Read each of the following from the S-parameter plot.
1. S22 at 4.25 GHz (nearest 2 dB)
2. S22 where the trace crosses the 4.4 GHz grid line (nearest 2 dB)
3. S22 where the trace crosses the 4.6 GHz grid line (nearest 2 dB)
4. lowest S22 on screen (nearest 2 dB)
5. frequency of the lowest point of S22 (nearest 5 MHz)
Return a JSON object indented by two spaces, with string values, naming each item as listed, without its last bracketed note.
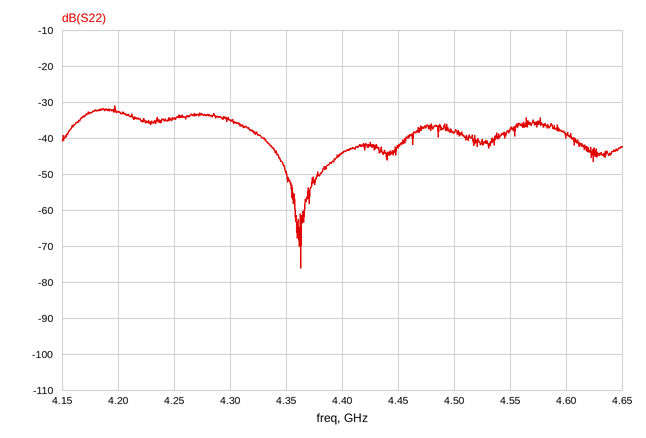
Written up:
{
  "S22 at 4.25 GHz": "-34 dB",
  "S22 where the trace crosses the 4.4 GHz grid line": "-44 dB",
  "S22 where the trace crosses the 4.6 GHz grid line": "-40 dB",
  "lowest S22 on screen": "-76 dB",
  "frequency of the lowest point of S22": "4.365 GHz"
}
